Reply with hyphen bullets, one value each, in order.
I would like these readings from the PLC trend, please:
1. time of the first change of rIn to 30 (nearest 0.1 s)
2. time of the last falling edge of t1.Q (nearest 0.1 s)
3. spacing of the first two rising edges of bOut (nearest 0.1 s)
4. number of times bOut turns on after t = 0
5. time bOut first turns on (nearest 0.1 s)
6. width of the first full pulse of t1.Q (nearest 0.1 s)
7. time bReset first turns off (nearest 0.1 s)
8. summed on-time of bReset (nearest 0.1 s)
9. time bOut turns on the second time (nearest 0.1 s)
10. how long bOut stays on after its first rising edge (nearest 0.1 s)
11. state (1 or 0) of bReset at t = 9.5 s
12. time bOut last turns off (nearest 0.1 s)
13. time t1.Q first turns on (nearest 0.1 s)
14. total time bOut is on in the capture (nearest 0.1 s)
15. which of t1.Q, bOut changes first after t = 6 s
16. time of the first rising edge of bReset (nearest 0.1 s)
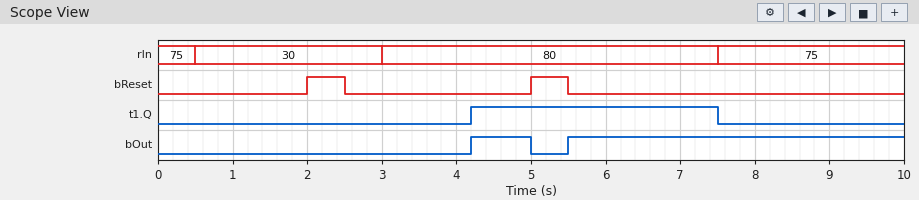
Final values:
- 0.5 s
- 7.5 s
- 1.3 s
- 2
- 4.2 s
- 3.3 s
- 2.5 s
- 1.0 s
- 5.5 s
- 0.8 s
- 0
- 5.0 s
- 4.2 s
- 5.3 s
- t1.Q
- 2.0 s
